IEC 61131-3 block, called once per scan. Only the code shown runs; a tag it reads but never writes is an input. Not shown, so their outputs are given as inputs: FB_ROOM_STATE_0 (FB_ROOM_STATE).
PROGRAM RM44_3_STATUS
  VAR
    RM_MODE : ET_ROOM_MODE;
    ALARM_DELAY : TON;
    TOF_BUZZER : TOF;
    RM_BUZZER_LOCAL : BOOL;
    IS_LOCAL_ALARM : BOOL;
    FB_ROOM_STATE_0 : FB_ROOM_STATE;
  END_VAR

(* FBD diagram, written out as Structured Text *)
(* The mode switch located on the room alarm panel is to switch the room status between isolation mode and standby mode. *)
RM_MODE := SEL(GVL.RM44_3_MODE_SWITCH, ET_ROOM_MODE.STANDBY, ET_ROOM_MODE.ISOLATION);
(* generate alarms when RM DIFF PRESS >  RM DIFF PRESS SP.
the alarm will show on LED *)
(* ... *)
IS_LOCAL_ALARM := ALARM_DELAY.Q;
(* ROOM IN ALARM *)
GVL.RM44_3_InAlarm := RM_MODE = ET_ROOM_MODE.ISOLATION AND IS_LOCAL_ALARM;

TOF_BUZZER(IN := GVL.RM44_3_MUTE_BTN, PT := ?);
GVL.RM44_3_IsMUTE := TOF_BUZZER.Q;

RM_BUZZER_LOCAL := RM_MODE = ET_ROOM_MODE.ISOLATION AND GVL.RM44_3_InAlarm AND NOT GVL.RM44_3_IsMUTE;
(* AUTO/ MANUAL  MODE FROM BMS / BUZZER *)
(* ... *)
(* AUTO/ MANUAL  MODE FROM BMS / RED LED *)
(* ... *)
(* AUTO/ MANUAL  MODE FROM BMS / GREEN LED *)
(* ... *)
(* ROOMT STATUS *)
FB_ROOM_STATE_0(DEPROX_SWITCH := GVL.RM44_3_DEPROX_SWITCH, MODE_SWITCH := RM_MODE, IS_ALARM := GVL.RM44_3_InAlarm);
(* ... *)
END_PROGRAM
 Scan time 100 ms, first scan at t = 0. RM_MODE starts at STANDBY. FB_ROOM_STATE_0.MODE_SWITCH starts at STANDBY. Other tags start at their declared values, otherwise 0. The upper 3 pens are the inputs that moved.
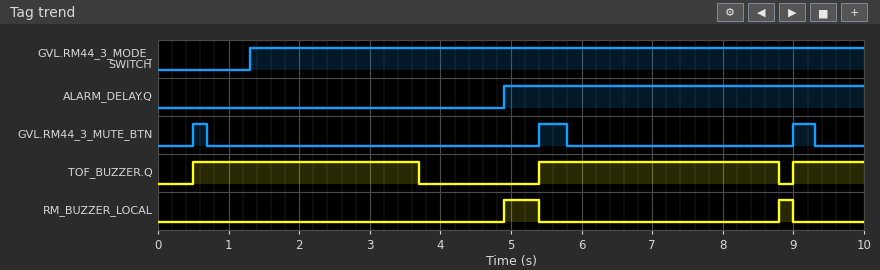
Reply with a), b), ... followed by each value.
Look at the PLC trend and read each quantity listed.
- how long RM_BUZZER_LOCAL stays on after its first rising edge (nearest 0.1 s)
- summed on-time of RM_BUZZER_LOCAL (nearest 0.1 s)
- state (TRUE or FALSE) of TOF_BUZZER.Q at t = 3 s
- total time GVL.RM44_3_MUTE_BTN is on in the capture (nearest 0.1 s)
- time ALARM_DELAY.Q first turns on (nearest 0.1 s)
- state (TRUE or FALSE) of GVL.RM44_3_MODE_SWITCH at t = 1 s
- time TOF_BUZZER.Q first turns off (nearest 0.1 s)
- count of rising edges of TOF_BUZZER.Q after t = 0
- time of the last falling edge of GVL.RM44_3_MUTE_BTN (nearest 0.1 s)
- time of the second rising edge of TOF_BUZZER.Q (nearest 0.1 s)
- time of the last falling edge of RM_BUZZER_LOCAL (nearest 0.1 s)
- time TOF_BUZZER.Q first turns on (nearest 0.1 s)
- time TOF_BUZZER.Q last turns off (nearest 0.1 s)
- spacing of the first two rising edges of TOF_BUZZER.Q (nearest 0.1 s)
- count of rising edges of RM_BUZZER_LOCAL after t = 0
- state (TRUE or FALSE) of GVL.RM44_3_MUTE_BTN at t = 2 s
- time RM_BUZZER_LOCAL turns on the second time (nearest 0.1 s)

a) 0.5 s
b) 0.7 s
c) TRUE
d) 0.9 s
e) 4.9 s
f) FALSE
g) 3.7 s
h) 3
i) 9.3 s
j) 5.4 s
k) 9.0 s
l) 0.5 s
m) 8.8 s
n) 4.9 s
o) 2
p) FALSE
q) 8.8 s
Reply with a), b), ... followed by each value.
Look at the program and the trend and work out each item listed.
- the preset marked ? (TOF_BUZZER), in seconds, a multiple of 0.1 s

a) 3.0 s
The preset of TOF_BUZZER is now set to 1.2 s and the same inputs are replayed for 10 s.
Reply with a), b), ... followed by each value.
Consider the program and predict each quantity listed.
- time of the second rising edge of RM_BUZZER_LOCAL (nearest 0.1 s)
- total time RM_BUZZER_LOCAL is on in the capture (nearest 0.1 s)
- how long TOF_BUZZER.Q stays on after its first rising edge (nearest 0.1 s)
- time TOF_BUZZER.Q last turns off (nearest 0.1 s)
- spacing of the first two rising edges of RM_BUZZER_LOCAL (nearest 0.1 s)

a) 7.0 s
b) 2.5 s
c) 1.4 s
d) 7.0 s
e) 2.1 s
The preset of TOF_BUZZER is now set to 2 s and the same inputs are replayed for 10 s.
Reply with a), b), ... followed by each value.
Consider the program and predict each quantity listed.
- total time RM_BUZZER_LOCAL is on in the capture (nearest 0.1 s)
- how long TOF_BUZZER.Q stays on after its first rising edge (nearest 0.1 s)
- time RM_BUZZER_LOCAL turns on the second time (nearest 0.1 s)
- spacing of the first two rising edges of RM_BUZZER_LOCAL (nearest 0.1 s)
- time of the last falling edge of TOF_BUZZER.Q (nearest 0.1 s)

a) 1.7 s
b) 2.2 s
c) 7.8 s
d) 2.9 s
e) 7.8 s
